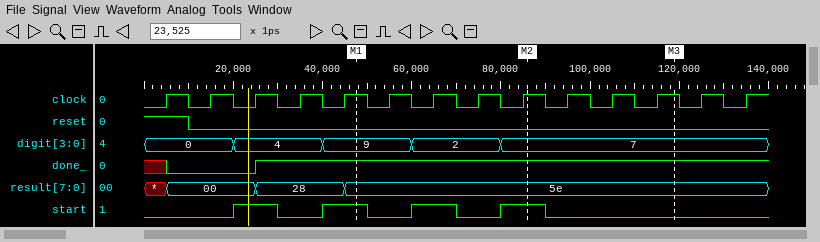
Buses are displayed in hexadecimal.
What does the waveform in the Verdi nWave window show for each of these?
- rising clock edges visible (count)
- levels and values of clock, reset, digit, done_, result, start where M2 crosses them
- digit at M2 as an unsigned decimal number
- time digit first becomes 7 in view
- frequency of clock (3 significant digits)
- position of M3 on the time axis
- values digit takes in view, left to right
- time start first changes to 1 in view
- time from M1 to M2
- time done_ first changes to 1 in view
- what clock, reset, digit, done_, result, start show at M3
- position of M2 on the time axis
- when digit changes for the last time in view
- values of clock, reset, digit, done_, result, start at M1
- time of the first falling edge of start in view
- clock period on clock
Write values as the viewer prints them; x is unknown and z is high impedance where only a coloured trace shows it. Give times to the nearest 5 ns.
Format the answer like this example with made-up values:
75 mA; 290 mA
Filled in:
14; clock=1, reset=0, digit=7, done_=1, result=5e, start=1; 7; 80 ns; 100 MHz; 120 ns; 0, 4, 9, 2, 7; 20 ns; 40 ns; 25 ns; clock=1, reset=0, digit=7, done_=1, result=5e, start=0; 85 ns; 80 ns; clock=1, reset=0, digit=9, done_=1, result=5e, start=1; 30 ns; 10 ns
